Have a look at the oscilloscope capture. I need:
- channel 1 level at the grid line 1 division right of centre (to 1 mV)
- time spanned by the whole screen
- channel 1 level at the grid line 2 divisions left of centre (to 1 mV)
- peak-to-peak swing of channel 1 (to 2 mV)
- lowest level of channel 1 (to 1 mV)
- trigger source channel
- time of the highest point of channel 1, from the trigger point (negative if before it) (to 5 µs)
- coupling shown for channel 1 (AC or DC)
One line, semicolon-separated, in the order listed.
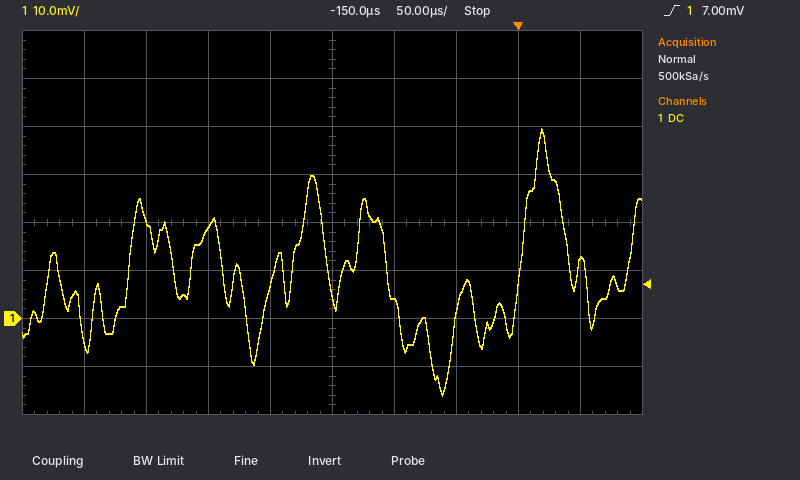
4 mV; 500 µs; 19 mV; 56 mV; -16 mV; channel 1; +20 µs; DC
